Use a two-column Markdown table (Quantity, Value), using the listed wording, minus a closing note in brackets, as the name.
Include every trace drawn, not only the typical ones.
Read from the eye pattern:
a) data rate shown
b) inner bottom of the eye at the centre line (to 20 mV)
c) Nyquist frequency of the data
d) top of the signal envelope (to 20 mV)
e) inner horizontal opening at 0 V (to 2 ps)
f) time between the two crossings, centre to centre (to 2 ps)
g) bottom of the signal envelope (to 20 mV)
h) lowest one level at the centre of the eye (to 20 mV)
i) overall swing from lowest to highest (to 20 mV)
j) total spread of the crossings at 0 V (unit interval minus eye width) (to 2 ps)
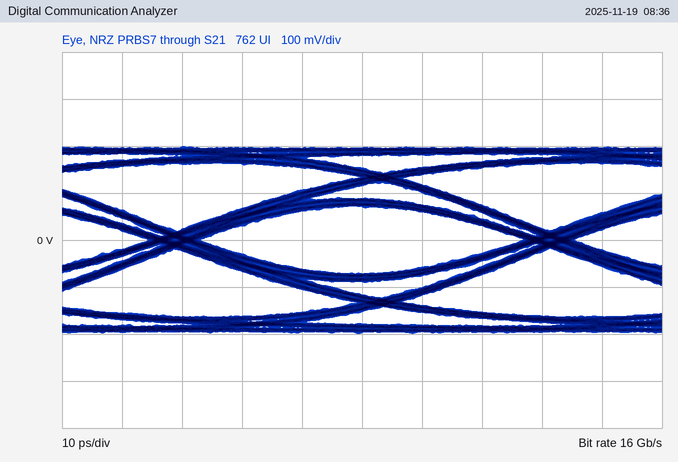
| Quantity | Value |
|---|---|
| data rate shown | 16 Gb/s |
| inner bottom of the eye at the centre line | -80 mV |
| Nyquist frequency of the data | 8 GHz |
| top of the signal envelope | 200 mV |
| inner horizontal opening at 0 V | 54 ps |
| time between the two crossings, centre to centre | 62 ps |
| bottom of the signal envelope | -200 mV |
| lowest one level at the centre of the eye | 80 mV |
| overall swing from lowest to highest | 400 mV |
| total spread of the crossings at 0 V (unit interval minus eye width) | 8 ps |
